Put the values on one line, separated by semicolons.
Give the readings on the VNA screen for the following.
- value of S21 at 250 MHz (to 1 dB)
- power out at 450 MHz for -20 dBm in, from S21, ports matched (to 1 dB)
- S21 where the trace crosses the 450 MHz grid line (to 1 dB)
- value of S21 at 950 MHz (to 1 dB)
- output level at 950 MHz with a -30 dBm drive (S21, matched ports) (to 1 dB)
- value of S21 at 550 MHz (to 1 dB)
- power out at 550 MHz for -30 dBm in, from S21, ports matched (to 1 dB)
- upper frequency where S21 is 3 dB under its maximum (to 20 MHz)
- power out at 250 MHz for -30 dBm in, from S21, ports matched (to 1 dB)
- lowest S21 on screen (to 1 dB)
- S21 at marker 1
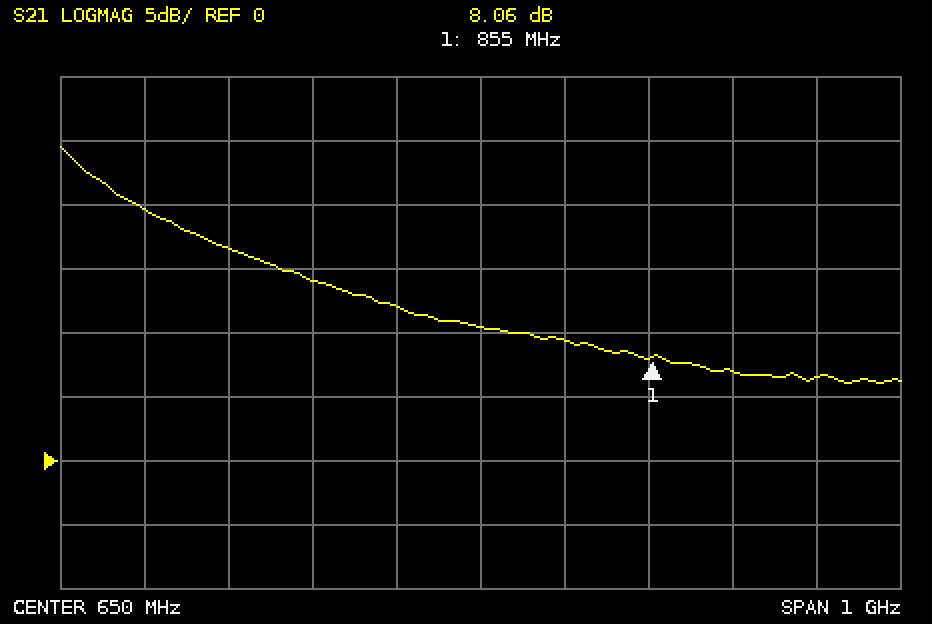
20 dB; -6 dBm; 14 dB; 7 dB; -23 dBm; 12 dB; -18 dBm; 200 MHz; -10 dBm; 6 dB; 8.06 dB
